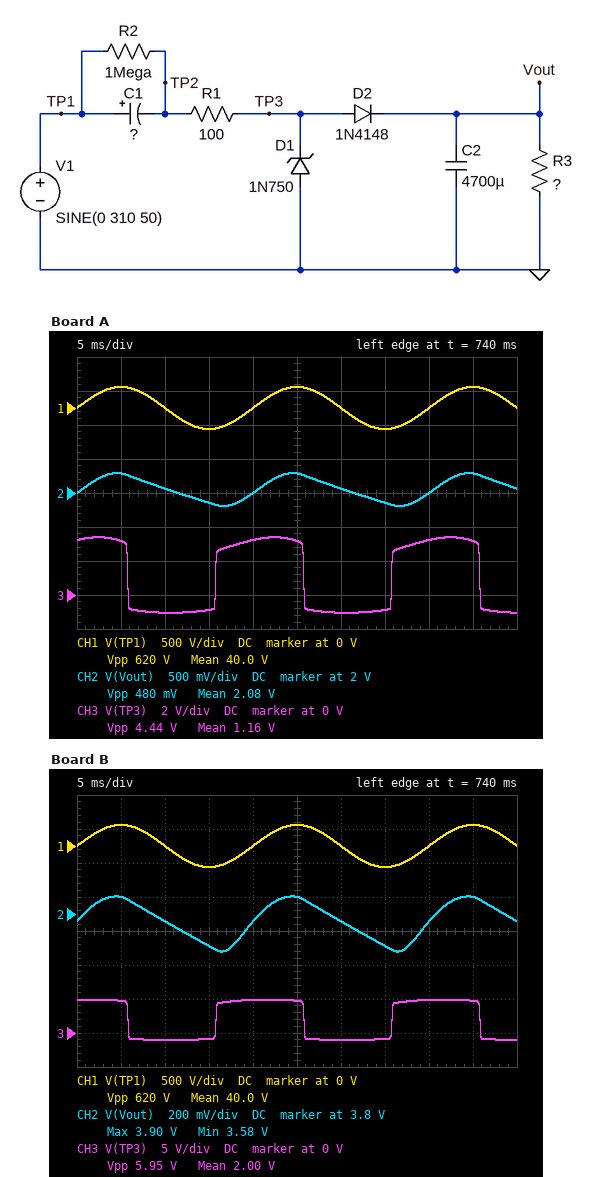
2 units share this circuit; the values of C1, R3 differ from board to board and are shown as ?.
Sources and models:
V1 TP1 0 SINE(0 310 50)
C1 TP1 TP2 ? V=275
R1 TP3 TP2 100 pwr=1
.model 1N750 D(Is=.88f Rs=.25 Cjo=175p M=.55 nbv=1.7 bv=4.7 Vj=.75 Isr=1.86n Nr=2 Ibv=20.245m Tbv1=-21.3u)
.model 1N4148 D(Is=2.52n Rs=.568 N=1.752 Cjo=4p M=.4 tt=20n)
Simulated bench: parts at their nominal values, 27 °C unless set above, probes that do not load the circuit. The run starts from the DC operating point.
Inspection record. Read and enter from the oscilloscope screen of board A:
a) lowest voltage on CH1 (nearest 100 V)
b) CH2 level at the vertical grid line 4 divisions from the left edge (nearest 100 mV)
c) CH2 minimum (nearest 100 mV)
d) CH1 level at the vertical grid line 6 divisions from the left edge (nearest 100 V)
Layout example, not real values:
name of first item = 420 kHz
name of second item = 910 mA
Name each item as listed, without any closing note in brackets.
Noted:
lowest voltage on CH1 = -300 V
CH2 level at the vertical grid line 4 divisions from the left edge = 2.0 V
CH2 minimum = 1.8 V
CH1 level at the vertical grid line 6 divisions from the left edge = 0 V
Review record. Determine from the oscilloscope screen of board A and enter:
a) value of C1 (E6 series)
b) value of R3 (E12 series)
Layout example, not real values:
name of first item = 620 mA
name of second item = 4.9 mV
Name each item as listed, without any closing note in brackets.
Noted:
value of C1 = 6.8 µF
value of R3 = 10 Ω
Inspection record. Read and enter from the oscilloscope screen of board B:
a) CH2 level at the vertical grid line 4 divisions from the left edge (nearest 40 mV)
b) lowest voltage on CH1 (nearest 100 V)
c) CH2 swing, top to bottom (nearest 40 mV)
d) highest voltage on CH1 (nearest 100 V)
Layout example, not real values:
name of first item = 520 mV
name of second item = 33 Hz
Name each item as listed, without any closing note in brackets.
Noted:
CH2 level at the vertical grid line 4 divisions from the left edge = 3.76 V
lowest voltage on CH1 = -300 V
CH2 swing, top to bottom = 320 mV
highest voltage on CH1 = 300 V
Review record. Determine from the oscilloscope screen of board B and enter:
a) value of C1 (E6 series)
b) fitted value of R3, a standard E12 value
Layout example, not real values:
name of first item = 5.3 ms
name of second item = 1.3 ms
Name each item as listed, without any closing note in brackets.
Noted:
value of C1 = 6.8 µF
fitted value of R3, a standard E12 value = 27 Ω
